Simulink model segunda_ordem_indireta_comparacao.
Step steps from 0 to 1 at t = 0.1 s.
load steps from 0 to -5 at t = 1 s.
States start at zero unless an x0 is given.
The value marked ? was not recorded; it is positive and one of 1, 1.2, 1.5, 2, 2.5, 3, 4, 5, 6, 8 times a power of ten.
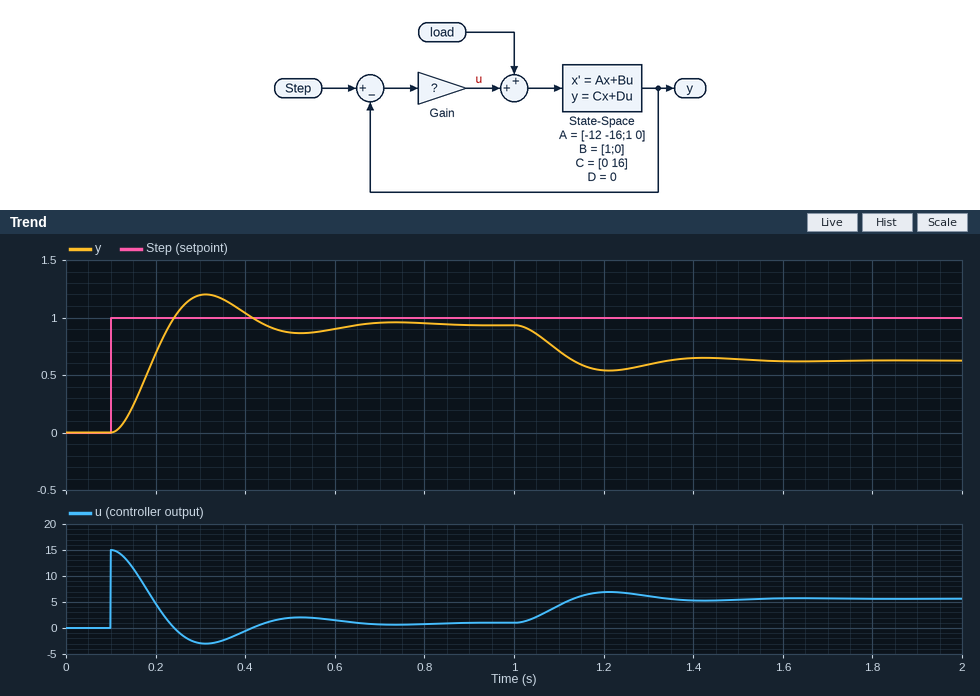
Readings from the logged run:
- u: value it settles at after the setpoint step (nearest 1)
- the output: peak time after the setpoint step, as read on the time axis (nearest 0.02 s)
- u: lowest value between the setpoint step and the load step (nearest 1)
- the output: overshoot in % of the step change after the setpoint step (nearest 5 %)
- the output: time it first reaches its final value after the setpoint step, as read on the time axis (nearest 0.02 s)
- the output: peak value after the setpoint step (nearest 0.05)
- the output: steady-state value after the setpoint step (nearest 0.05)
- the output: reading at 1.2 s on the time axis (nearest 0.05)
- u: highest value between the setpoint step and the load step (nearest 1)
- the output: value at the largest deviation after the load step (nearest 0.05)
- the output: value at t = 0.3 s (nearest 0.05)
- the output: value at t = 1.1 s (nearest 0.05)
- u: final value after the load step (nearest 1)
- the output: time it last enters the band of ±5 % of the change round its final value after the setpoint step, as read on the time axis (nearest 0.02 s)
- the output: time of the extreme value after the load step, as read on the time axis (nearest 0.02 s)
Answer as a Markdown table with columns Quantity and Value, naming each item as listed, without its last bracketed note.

| Quantity | Value |
|---|---|
| u: value it settles at after the setpoint step | 1 |
| the output: peak time after the setpoint step, as read on the time axis | 0.32 s |
| u: lowest value between the setpoint step and the load step | -3 |
| the output: overshoot in % of the step change after the setpoint step | 30 % |
| the output: time it first reaches its final value after the setpoint step, as read on the time axis | 0.24 s |
| the output: peak value after the setpoint step | 1.20 |
| the output: steady-state value after the setpoint step | 0.95 |
| the output: reading at 1.2 s on the time axis | 0.55 |
| u: highest value between the setpoint step and the load step | 15 |
| the output: value at the largest deviation after the load step | 0.55 |
| the output: value at t = 0.3 s | 1.20 |
| the output: value at t = 1.1 s | 0.70 |
| u: final value after the load step | 6 |
| the output: time it last enters the band of ±5 % of the change round its final value after the setpoint step, as read on the time axis | 0.58 s |
| the output: time of the extreme value after the load step, as read on the time axis | 1.22 s |
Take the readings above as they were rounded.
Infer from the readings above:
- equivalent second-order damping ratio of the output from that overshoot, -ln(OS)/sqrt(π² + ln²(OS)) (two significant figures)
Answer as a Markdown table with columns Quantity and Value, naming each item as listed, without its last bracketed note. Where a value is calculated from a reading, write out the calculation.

| Quantity | Value |
|---|---|
| equivalent second-order damping ratio of the output from that overshoot, -ln(OS)/sqrt(π² + ln²(OS)) | ln(0.3) = -1.204; 1.204 / sqrt(9.870 + 1.450) = 0.36 |
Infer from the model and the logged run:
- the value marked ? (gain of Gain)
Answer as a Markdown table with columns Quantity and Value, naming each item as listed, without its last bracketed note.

| Quantity | Value |
|---|---|
| the value marked ? | 15 |
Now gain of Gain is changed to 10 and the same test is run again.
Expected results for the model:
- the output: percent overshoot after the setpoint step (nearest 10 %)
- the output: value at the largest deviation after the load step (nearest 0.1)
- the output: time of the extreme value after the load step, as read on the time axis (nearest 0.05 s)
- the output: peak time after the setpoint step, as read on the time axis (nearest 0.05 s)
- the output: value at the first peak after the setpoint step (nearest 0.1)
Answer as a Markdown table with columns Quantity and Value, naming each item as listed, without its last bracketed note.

| Quantity | Value |
|---|---|
| the output: percent overshoot after the setpoint step | 20 % |
| the output: value at the largest deviation after the load step | 0.4 |
| the output: time of the extreme value after the load step, as read on the time axis | 1.25 s |
| the output: peak time after the setpoint step, as read on the time axis | 0.35 s |
| the output: value at the first peak after the setpoint step | 1.1 |
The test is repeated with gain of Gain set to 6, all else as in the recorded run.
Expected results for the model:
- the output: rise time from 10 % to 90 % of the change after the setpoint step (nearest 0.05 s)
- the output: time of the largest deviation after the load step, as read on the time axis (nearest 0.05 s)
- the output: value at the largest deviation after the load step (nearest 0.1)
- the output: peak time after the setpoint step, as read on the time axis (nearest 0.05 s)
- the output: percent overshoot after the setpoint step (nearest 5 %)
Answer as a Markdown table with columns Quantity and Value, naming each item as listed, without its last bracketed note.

| Quantity | Value |
|---|---|
| the output: rise time from 10 % to 90 % of the change after the setpoint step | 0.15 s |
| the output: time of the largest deviation after the load step, as read on the time axis | 1.35 s |
| the output: value at the largest deviation after the load step | 0.1 |
| the output: peak time after the setpoint step, as read on the time axis | 0.45 s |
| the output: percent overshoot after the setpoint step | 10 % |
